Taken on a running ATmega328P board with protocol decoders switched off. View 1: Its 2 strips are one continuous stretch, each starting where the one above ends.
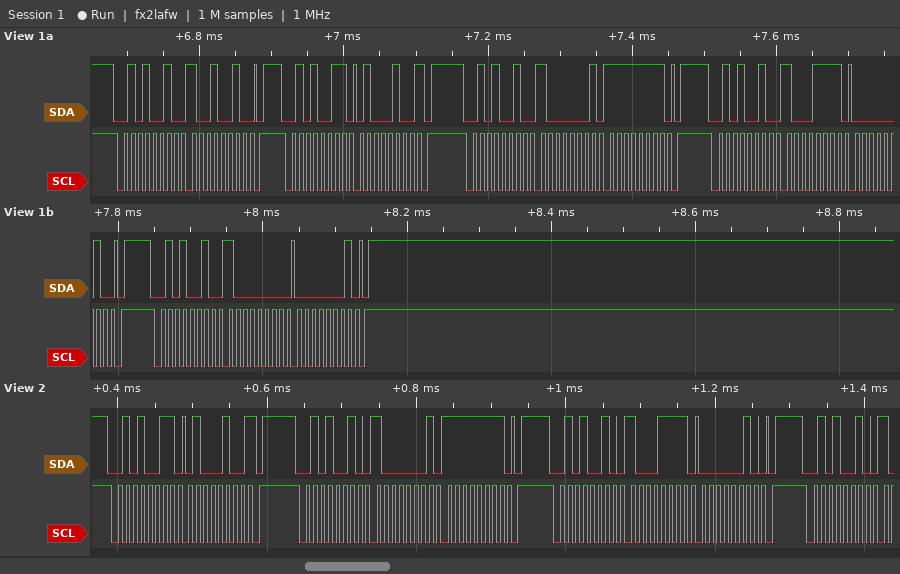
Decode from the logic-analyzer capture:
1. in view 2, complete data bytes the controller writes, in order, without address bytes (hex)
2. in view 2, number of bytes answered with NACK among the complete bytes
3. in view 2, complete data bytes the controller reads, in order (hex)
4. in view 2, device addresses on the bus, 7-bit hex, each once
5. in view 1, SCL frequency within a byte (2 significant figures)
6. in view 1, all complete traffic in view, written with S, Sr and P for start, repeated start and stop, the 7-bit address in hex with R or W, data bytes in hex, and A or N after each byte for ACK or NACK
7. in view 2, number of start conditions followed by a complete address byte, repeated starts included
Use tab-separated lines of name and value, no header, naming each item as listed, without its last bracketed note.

in view 2, complete data bytes the controller writes, in order, without address bytes	81 FF 8F 02
in view 2, number of bytes answered with NACK among the complete bytes	1
in view 2, complete data bytes the controller reads, in order	44
in view 2, device addresses on the bus, 7-bit hex, each once	0x29
in view 1, SCL frequency within a byte	100 kHz
in view 1, all complete traffic in view, written with S, Sr and P for start, repeated start and stop, the 7-bit address in hex with R or W, data bytes in hex, and A or N after each byte for ACK or NACK	S 29W A 92 A P S 29R A 44 N P S 29W A 81 A FF A P S 29W A 8F A 02 A P S 29W A 80 A 01 A P
in view 2, number of start conditions followed by a complete address byte, repeated starts included	4
